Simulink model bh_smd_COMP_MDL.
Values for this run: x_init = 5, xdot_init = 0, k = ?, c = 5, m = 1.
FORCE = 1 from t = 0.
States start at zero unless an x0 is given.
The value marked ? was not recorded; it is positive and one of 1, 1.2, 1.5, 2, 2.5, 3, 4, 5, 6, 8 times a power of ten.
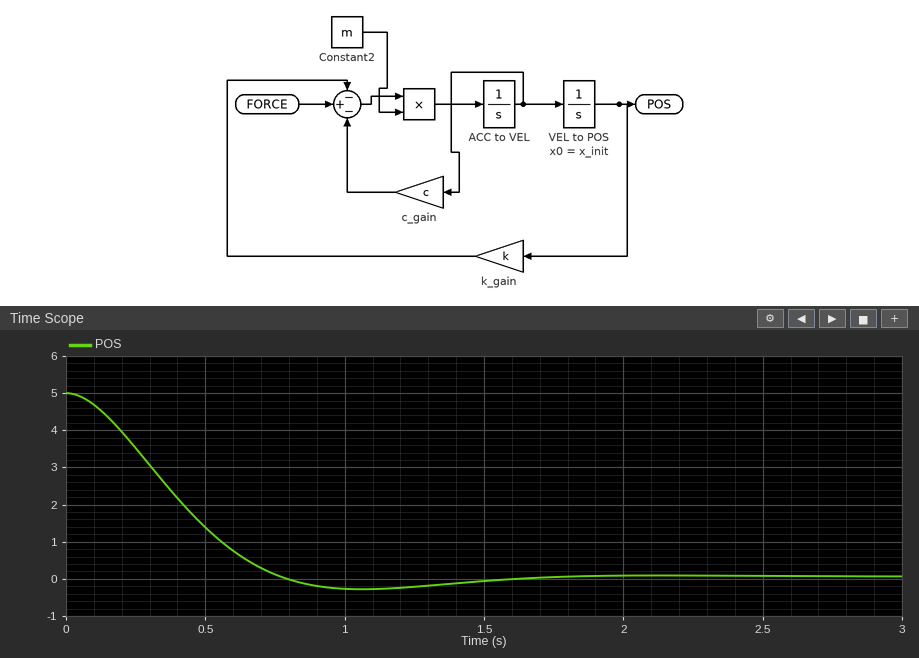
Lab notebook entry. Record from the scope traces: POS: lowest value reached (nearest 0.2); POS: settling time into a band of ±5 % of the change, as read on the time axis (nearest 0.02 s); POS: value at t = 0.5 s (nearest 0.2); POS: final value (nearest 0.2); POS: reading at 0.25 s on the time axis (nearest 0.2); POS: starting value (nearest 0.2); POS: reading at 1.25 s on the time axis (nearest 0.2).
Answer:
-0.2
1.30 s
1.4
0.0
3.6
5.0
-0.2
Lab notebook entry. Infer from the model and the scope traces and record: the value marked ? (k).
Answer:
15
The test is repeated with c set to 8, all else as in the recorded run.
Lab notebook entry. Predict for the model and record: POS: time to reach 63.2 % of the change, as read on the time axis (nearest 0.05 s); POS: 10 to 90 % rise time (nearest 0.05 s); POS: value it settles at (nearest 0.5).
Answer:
0.55 s
0.90 s
0.0
